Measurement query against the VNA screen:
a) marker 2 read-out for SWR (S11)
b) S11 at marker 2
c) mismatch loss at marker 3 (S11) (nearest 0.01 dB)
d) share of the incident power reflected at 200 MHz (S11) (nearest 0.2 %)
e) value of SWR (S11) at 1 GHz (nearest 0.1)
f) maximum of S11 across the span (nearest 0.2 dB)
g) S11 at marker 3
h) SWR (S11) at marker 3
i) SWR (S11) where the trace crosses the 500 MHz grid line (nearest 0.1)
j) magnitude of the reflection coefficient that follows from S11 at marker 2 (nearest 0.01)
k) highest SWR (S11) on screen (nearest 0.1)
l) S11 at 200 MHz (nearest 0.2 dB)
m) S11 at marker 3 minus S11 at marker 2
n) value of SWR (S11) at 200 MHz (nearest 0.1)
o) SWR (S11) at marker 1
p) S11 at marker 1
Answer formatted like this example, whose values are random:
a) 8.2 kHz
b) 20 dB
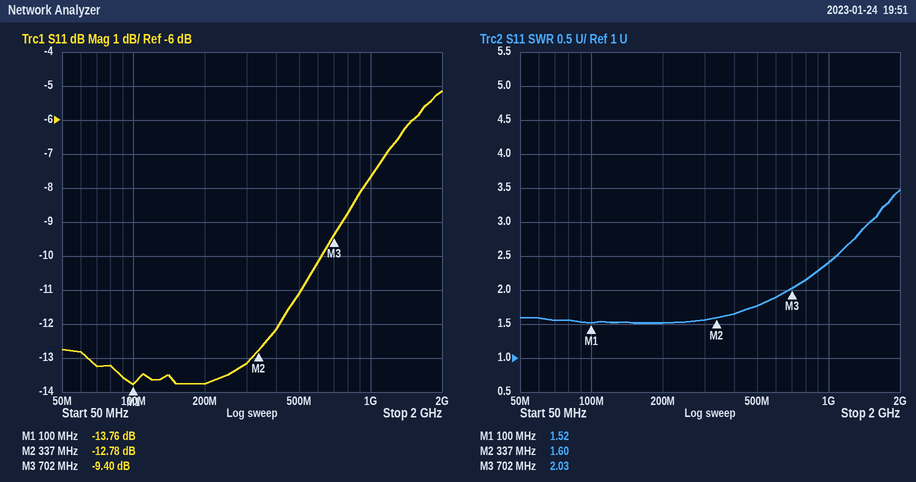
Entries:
a) 1.60
b) -12.78 dB
c) 0.53 dB
d) 4.2 %
e) 2.4
f) -5.2 dB
g) -9.40 dB
h) 2.03
i) 1.8
j) 0.23
k) 3.5
l) -13.8 dB
m) 3.38 dB
n) 1.5
o) 1.52
p) -13.76 dB
